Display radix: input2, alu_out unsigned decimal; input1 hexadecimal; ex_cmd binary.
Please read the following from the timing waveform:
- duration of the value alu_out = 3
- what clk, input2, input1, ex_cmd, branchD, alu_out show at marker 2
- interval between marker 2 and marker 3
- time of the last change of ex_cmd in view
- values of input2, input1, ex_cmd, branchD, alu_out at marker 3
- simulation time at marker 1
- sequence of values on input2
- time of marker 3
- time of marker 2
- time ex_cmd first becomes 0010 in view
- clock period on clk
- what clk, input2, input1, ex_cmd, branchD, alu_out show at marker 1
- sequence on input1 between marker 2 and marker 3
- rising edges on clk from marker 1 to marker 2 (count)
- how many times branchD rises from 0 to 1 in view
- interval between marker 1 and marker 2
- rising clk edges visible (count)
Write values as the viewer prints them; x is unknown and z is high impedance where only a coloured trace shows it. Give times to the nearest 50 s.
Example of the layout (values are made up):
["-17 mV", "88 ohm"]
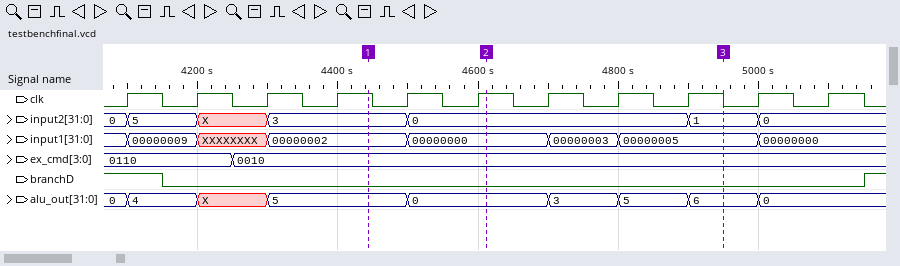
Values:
["100 s", "clk=1, input2=0, input1=00000000, ex_cmd=0010, branchD=0, alu_out=0", "350 s", "4250 s", "input2=1, input1=00000005, ex_cmd=0010, branchD=0, alu_out=6", "4450 s", "0, 5, X, 3, 0, 1, 0", "4950 s", "4600 s", "4250 s", "100 s", "clk=1, input2=3, input1=00000002, ex_cmd=0010, branchD=0, alu_out=5", "00000000, 00000003, 00000005", "2", "1", "150 s", "11"]
